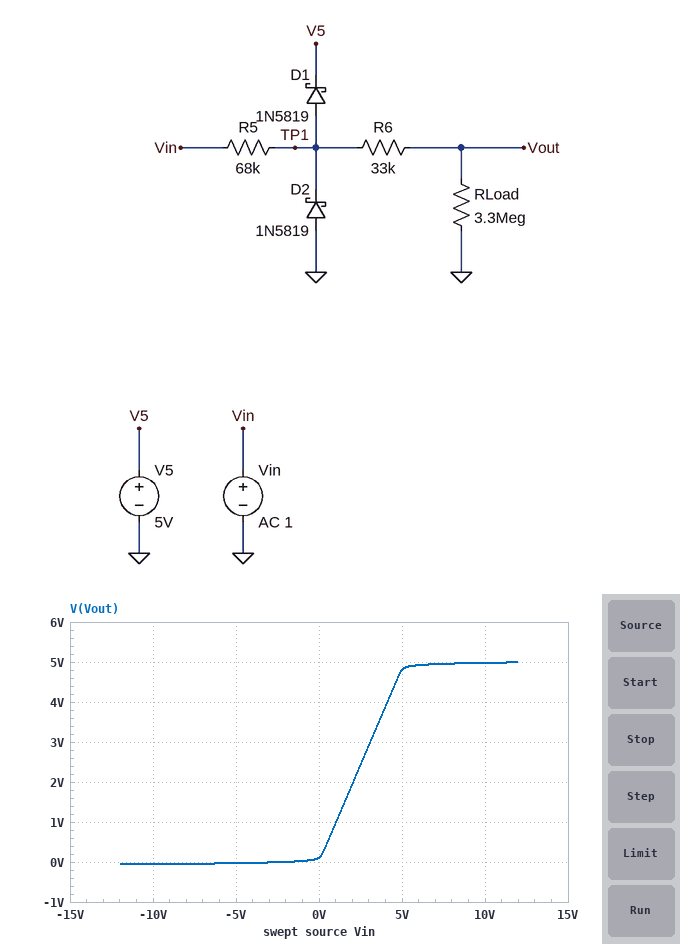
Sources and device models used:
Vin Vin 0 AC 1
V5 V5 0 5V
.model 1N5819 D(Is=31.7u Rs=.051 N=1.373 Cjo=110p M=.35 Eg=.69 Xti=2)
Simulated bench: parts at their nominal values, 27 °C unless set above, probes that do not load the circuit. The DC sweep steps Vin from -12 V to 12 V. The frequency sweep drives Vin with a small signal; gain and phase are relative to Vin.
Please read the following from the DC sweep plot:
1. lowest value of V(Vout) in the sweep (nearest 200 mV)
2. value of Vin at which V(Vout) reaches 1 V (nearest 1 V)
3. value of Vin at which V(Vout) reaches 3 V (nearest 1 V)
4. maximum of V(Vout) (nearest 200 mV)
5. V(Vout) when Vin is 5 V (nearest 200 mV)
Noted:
0 V
1 V
3 V
5.0 V
4.8 V
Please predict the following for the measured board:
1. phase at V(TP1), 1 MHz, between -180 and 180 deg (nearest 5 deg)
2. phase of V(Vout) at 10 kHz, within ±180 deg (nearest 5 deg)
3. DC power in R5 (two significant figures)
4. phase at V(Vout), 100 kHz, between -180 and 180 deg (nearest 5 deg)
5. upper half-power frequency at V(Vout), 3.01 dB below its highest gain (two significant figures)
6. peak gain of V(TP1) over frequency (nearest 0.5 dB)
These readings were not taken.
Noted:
-85 deg
-10 deg
170 nW
-60 deg
58 kHz
-12.0 dB
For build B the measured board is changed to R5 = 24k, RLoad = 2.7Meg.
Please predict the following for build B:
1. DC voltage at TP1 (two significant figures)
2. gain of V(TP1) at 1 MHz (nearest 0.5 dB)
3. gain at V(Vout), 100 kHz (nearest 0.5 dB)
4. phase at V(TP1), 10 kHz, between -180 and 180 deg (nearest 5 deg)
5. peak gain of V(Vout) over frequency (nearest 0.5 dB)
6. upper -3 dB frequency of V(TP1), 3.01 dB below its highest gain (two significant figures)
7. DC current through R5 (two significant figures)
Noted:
80 mV
-28.0 dB
-12.5 dB
-5 deg
-10.5 dB
130 kHz
3.3 µA
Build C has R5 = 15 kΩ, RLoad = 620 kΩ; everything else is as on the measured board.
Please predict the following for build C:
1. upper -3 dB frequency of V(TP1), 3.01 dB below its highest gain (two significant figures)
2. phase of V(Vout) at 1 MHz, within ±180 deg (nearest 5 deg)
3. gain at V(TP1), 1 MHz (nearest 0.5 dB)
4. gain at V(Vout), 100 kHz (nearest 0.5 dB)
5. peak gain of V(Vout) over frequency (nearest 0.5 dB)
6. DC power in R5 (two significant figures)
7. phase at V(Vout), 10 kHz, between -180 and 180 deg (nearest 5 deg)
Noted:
190 kHz
-80 deg
-24.0 dB
-11.0 dB
-10.0 dB
310 nW
-5 deg
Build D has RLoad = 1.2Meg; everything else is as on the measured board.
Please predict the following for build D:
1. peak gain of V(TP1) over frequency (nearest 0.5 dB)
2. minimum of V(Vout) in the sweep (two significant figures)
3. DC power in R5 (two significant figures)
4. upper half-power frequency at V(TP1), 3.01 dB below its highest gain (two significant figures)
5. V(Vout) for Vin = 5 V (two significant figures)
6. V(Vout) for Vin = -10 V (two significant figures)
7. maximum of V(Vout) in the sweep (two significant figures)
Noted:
-12.5 dB
-59 mV
160 nW
59 kHz
4.6 V
-53 mV
4.9 V
